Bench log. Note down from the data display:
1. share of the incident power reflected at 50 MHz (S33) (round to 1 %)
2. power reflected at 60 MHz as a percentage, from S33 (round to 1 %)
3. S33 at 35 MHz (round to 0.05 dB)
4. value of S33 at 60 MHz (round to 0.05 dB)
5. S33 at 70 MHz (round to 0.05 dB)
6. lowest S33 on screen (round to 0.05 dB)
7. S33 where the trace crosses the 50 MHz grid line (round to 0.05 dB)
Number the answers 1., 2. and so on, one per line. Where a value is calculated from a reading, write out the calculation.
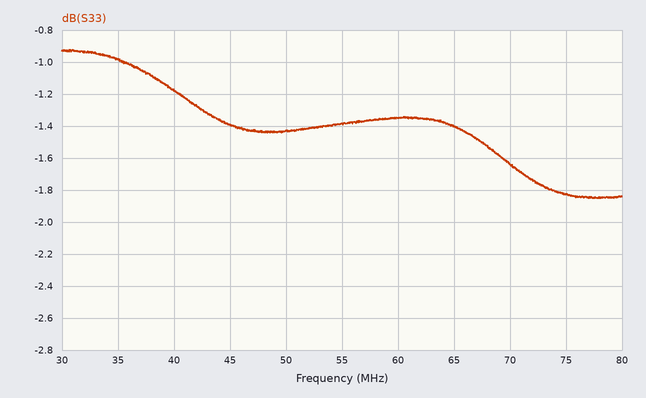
1. 10^(-1.45/10) ≈ 72 %
2. 10^(-1.35/10) ≈ 73 %
3. -1.00 dB
4. -1.35 dB
5. -1.65 dB
6. -1.85 dB
7. -1.45 dB
